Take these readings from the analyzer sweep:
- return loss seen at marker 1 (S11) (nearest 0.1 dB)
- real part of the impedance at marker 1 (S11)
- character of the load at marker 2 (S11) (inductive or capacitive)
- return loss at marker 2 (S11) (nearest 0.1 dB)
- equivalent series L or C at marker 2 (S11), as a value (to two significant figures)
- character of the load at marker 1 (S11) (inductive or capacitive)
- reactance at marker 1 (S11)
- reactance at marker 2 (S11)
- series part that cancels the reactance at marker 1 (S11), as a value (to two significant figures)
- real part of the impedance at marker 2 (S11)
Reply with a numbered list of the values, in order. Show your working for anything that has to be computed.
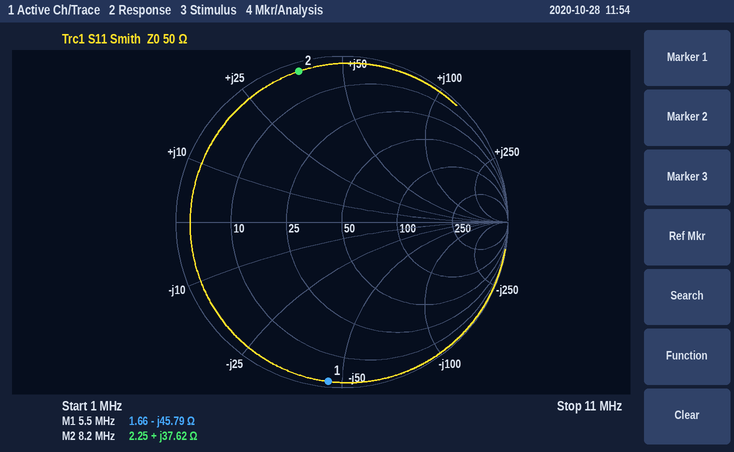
1. 0.3 dB
2. 1.66 Ω
3. inductive
4. 0.5 dB
5. L = 37.62 Ω/(2π × 8.2 MHz) ≈ 730 nH
6. capacitive
7. -45.79 Ω
8. +37.62 Ω
9. L = 45.79 Ω/(2π × 5.5 MHz) ≈ 1.3 µH
10. 2.25 Ω
